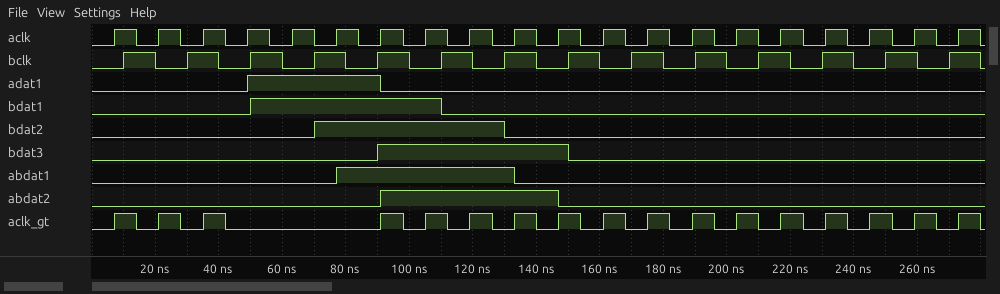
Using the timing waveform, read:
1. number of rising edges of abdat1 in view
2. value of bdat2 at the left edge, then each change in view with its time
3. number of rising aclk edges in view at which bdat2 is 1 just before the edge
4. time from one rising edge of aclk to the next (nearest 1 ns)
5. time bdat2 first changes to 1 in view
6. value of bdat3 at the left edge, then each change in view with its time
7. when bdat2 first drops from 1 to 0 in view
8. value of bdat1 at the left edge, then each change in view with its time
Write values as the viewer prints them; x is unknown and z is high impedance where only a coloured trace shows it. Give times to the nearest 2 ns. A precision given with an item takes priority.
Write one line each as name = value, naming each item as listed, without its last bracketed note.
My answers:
number of rising edges of abdat1 in view = 1
value of bdat2 at the left edge, then each change in view with its time = 0, 1 at 70 ns, 0 at 130 ns
number of rising aclk edges in view at which bdat2 is 1 just before the edge = 4
time from one rising edge of aclk to the next = 14 ns
time bdat2 first changes to 1 in view = 70 ns
value of bdat3 at the left edge, then each change in view with its time = 0, 1 at 90 ns, 0 at 150 ns
when bdat2 first drops from 1 to 0 in view = 130 ns
value of bdat1 at the left edge, then each change in view with its time = 0, 1 at 50 ns, 0 at 110 ns
